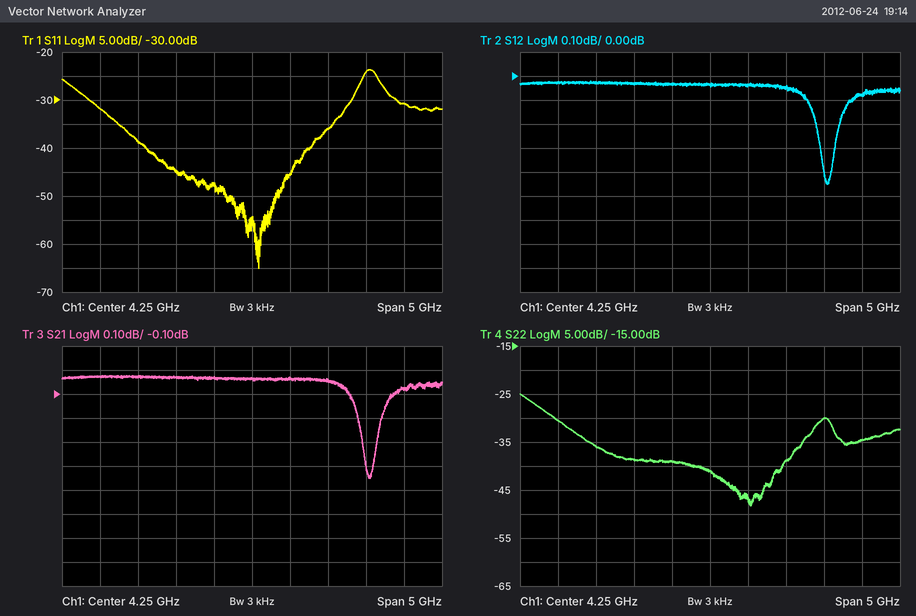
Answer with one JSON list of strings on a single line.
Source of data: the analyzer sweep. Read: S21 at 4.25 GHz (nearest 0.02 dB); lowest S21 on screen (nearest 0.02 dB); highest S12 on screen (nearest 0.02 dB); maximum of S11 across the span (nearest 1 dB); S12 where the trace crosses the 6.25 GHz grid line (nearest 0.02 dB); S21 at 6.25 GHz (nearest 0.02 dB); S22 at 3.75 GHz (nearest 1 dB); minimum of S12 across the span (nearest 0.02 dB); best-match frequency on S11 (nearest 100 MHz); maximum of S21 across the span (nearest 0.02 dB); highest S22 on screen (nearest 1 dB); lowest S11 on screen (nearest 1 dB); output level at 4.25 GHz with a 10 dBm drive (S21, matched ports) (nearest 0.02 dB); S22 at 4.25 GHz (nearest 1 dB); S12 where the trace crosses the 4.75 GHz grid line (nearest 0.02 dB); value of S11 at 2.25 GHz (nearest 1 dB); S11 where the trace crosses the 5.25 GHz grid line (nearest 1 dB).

["-0.04 dB", "-0.46 dB", "-0.02 dB", "-24 dB", "-0.08 dB", "-0.08 dB", "-39 dB", "-0.46 dB", "4.3 GHz", "-0.02 dB", "-25 dB", "-65 dB", "9.96 dBm", "-41 dB", "-0.04 dB", "-32 dB", "-36 dB"]
